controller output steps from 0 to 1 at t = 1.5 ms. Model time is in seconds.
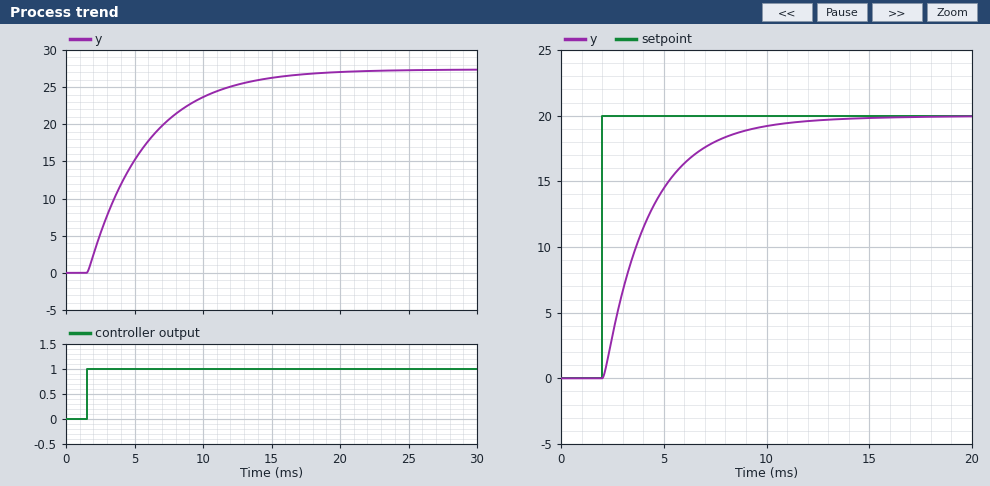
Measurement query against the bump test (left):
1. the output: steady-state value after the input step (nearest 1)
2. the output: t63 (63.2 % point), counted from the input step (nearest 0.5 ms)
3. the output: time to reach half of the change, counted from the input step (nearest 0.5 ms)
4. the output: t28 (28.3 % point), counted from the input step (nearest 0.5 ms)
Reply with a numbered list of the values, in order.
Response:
1. 27
2. 4.5 ms
3. 3.0 ms
4. 1.5 ms
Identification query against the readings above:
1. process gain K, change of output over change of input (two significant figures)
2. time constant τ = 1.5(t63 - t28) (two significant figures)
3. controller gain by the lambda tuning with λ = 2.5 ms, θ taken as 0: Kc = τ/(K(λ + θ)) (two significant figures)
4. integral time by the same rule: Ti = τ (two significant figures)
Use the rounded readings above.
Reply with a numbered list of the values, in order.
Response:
1. 27
2. 4.5 ms
3. 0.067
4. 4.5 ms
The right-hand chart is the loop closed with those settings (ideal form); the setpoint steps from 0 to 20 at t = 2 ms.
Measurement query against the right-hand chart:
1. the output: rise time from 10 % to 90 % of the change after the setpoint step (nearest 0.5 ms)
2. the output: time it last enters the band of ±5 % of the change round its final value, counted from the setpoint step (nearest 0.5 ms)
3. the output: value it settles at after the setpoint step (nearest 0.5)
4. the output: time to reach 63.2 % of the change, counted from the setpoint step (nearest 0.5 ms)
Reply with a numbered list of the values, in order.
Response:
1. 5.0 ms
2. 7.5 ms
3. 20.0
4. 2.5 ms
